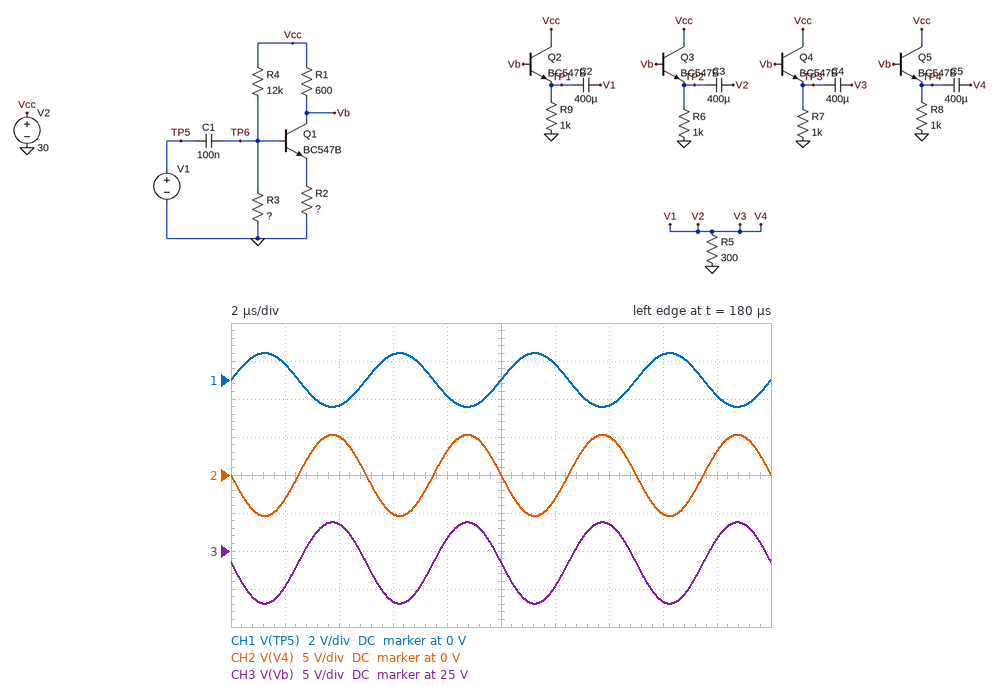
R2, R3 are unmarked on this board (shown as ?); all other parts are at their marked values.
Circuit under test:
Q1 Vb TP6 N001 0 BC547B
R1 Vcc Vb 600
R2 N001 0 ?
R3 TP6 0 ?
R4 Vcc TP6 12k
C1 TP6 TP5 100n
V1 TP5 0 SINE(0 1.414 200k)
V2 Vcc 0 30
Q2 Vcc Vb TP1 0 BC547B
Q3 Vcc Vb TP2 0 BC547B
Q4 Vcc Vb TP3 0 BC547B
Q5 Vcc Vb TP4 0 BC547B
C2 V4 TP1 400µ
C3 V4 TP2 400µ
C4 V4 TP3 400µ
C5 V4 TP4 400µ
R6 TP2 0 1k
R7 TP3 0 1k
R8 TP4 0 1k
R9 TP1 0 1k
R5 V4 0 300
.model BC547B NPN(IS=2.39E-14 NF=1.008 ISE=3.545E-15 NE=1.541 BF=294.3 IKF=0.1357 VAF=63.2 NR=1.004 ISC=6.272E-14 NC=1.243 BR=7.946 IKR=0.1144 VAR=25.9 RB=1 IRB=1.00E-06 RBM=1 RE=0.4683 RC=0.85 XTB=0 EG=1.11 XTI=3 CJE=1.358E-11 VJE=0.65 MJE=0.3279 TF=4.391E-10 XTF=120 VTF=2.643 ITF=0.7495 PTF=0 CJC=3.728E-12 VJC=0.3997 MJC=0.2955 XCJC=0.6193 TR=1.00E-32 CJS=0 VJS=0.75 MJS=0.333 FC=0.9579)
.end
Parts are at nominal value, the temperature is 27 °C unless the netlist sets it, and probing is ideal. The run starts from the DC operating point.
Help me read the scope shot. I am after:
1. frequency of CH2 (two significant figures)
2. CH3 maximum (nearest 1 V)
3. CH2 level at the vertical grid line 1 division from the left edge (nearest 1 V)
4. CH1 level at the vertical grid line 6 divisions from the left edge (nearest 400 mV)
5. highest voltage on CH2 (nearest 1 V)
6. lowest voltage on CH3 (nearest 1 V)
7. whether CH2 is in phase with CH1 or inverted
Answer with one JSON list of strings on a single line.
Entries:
["200 kHz", "29 V", "-3 V", "800 mV", "5 V", "18 V", "inverted"]
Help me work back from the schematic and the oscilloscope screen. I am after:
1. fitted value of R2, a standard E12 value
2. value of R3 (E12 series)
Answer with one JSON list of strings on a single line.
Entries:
["150 Ω", "1 kΩ"]
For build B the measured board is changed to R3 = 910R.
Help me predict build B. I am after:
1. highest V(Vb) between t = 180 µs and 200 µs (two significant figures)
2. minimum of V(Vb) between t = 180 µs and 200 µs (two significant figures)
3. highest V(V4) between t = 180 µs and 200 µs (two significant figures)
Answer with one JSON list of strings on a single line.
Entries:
["29 V", "19 V", "5.2 V"]
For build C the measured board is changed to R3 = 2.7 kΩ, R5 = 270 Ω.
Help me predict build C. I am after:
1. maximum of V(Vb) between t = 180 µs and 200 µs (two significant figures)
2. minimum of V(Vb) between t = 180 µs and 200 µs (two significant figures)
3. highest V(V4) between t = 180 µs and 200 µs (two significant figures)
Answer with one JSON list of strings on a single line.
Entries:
["17 V", "6.5 V", "5.5 V"]
